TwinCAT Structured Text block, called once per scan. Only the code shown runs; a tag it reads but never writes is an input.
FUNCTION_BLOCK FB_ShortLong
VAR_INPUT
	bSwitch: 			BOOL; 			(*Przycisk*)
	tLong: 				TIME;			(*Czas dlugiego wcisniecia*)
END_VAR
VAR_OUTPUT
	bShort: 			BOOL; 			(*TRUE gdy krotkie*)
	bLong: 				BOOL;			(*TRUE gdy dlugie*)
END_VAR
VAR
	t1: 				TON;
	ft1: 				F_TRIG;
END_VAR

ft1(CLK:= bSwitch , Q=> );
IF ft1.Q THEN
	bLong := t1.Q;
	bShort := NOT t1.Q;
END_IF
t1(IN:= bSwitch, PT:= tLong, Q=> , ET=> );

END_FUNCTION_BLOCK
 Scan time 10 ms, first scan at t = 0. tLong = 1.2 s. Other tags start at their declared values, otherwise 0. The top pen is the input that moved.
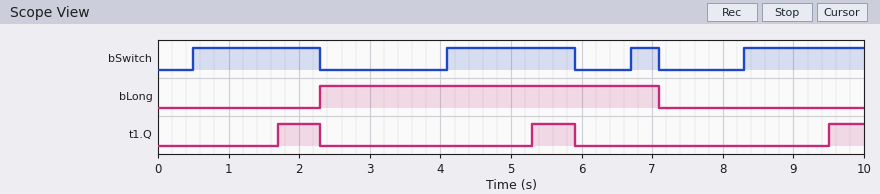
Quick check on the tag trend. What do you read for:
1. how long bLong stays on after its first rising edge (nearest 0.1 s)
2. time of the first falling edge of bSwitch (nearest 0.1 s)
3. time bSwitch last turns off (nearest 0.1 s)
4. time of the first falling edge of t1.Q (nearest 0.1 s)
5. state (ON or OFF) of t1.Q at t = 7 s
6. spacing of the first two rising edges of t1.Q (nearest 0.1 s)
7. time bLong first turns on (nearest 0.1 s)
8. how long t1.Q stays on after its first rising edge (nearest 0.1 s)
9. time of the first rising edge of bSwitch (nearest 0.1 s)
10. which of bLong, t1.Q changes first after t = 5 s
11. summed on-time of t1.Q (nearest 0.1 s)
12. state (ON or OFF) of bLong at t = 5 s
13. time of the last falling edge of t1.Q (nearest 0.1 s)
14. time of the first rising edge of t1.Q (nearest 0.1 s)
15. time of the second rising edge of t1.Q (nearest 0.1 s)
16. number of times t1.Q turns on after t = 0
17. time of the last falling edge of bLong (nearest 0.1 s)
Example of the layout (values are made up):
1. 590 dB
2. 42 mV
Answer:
1. 4.8 s
2. 2.3 s
3. 7.1 s
4. 2.3 s
5. OFF
6. 3.6 s
7. 2.3 s
8. 0.6 s
9. 0.5 s
10. t1.Q
11. 1.7 s
12. ON
13. 5.9 s
14. 1.7 s
15. 5.3 s
16. 3
17. 7.1 s
